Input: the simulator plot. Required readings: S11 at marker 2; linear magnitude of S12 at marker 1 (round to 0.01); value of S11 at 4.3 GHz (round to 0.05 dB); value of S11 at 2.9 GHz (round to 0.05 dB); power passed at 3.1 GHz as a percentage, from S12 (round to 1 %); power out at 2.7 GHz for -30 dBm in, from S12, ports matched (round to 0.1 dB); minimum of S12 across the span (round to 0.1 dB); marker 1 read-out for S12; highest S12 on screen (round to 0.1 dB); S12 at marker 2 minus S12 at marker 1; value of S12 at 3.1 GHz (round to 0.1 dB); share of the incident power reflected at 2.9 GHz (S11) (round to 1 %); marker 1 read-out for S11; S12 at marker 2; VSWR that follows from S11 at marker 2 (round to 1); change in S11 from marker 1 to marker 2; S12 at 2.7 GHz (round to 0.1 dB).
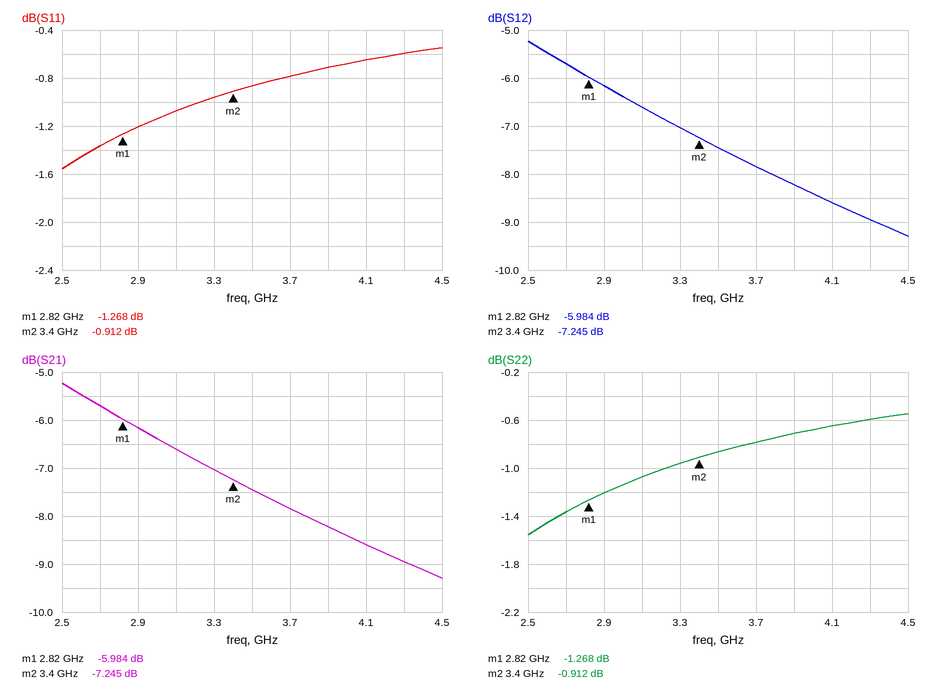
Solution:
-0.912 dB
0.50
-0.60 dB
-1.20 dB
22 %
-35.7 dBm
-9.3 dB
-5.984 dB
-5.2 dB
-1.261 dB
-6.6 dB
76 %
-1.268 dB
-7.245 dB
19
0.356 dB
-5.7 dB
